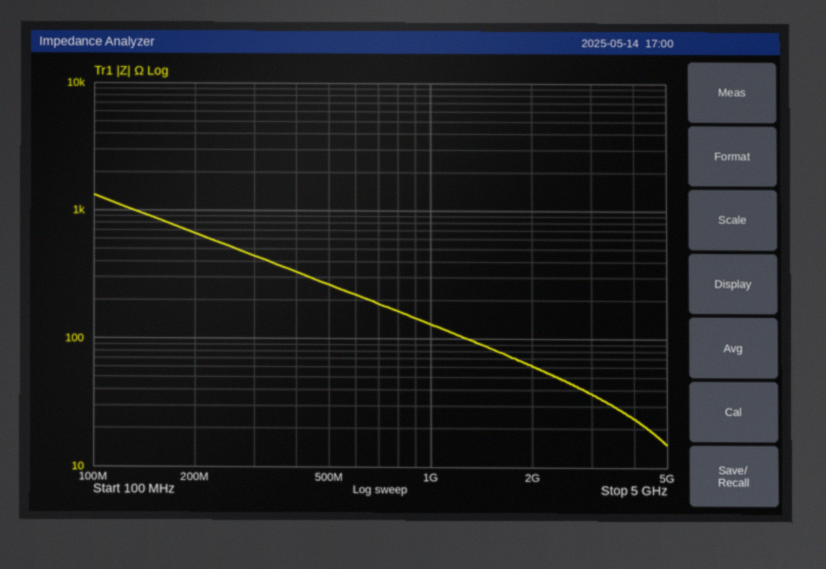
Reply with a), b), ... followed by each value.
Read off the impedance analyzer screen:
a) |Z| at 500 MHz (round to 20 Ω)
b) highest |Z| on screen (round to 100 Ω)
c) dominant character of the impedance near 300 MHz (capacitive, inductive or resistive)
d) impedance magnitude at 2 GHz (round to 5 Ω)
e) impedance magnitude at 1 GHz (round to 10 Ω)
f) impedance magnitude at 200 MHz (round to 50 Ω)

a) 260 Ω
b) 1.3 kΩ
c) capacitive
d) 60 Ω
e) 130 Ω
f) 650 Ω
